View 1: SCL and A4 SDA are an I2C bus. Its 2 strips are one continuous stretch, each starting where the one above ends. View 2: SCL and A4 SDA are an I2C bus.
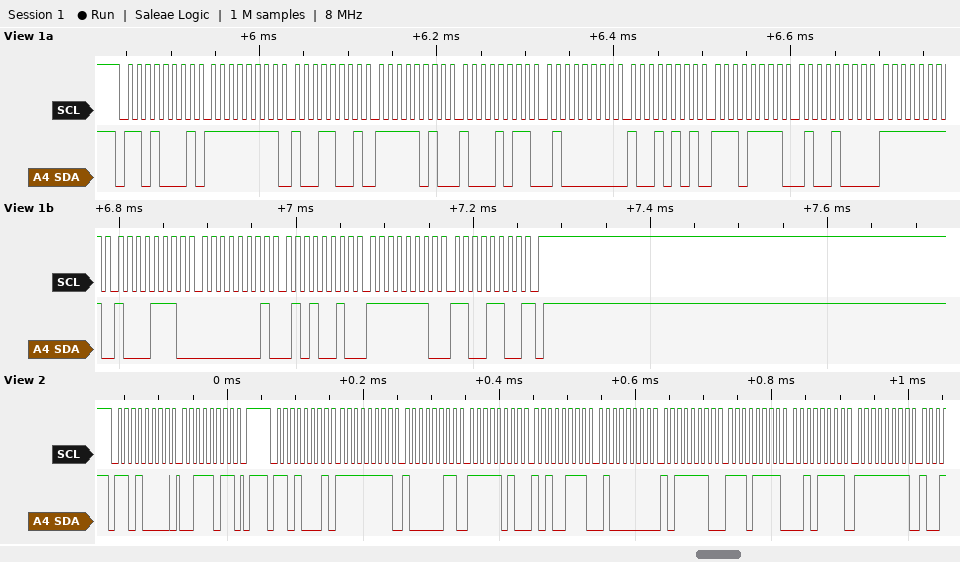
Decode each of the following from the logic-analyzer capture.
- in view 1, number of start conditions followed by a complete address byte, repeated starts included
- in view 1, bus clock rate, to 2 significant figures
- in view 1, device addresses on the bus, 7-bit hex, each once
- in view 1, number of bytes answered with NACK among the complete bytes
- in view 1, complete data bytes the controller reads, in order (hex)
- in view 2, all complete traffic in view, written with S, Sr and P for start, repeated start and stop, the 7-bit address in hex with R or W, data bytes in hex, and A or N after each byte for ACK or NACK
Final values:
1
100 kHz
0x68
1
FF 99 FA 8B 40 95 EF 48 FF 8E 01 52 FE CC
S 68W A 3B A P S 68R A FF A 83 A FA A A7 A 40 A BE A EF A 2F A FF A
